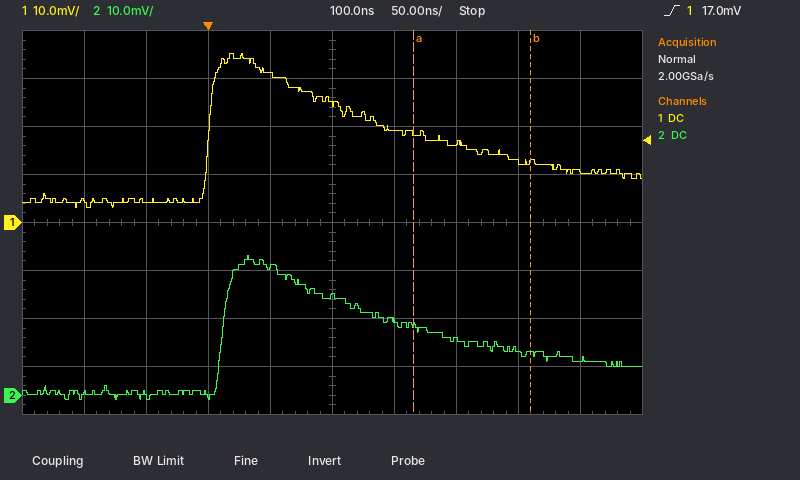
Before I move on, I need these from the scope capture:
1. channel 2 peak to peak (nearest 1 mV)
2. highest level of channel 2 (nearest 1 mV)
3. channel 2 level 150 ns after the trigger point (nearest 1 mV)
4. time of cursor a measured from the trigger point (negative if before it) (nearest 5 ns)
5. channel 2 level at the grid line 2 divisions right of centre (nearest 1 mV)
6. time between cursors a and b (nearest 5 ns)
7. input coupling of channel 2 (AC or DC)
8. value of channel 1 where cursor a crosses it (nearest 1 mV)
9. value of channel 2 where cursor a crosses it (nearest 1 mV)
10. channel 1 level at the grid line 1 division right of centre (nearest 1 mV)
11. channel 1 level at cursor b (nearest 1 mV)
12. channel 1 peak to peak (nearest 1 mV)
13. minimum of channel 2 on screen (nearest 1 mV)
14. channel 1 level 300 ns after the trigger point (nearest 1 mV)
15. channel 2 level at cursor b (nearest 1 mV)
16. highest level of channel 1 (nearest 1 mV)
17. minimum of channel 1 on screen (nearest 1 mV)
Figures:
30 mV
29 mV
16 mV
+165 ns
12 mV
95 ns
DC
19 mV
15 mV
19 mV
13 mV
32 mV
-1 mV
11 mV
9 mV
35 mV
3 mV
